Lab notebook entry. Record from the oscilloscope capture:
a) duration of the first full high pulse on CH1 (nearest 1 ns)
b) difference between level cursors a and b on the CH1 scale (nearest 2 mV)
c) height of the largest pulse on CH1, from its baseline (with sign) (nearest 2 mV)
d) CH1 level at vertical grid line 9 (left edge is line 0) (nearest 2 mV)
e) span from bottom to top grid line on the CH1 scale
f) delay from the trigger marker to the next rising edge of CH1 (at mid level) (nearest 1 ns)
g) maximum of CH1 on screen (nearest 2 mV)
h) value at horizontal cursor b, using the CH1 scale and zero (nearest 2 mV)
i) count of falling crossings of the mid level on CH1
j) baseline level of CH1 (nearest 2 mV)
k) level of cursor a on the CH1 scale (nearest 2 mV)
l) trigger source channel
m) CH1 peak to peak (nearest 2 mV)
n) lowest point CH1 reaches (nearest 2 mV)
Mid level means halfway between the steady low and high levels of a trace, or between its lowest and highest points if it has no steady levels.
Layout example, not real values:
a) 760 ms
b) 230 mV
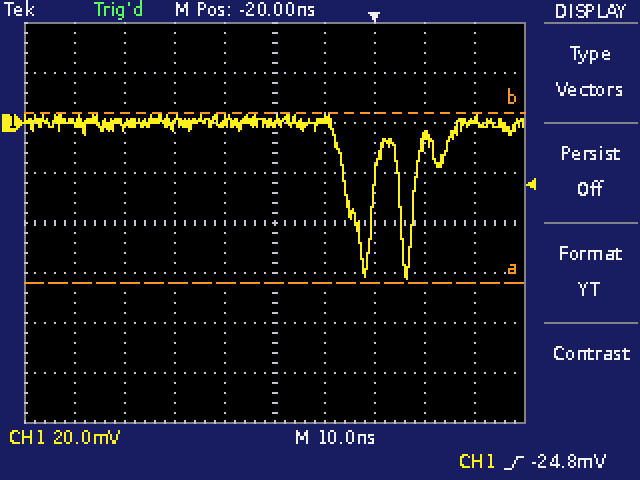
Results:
a) 5 ns
b) 68 mV
c) -62 mV
d) 2 mV
e) 160 mV
f) 8 ns
g) 4 mV
h) 4 mV
i) 2
j) 0 mV
k) -64 mV
l) CH1
m) 66 mV
n) -62 mV
